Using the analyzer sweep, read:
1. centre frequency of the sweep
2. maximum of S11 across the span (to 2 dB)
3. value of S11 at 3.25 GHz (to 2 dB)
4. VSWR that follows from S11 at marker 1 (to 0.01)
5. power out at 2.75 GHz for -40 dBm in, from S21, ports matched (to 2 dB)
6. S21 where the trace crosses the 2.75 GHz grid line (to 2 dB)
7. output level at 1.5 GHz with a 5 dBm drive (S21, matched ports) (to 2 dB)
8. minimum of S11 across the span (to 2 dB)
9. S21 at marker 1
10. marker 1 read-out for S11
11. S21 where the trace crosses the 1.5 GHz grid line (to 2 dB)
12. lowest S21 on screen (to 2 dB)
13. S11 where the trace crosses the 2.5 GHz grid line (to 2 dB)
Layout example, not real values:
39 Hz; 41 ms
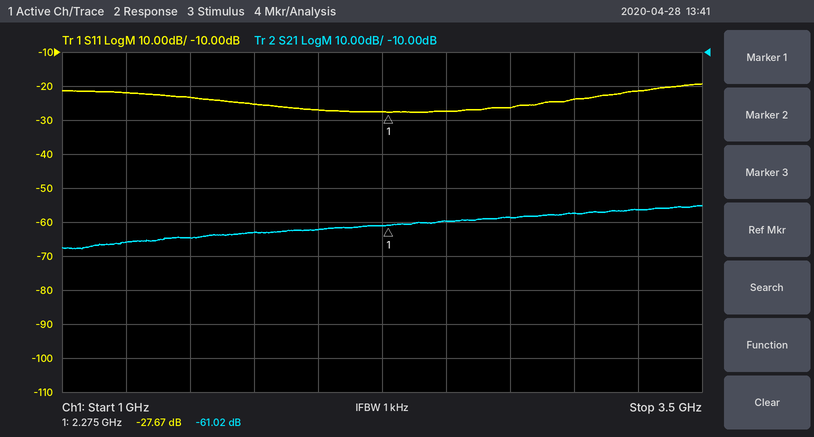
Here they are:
2.25 GHz; -20 dB; -22 dB; 1.09; -98 dBm; -58 dB; -60 dBm; -28 dB; -61.02 dB; -27.67 dB; -64 dB; -68 dB; -28 dB
